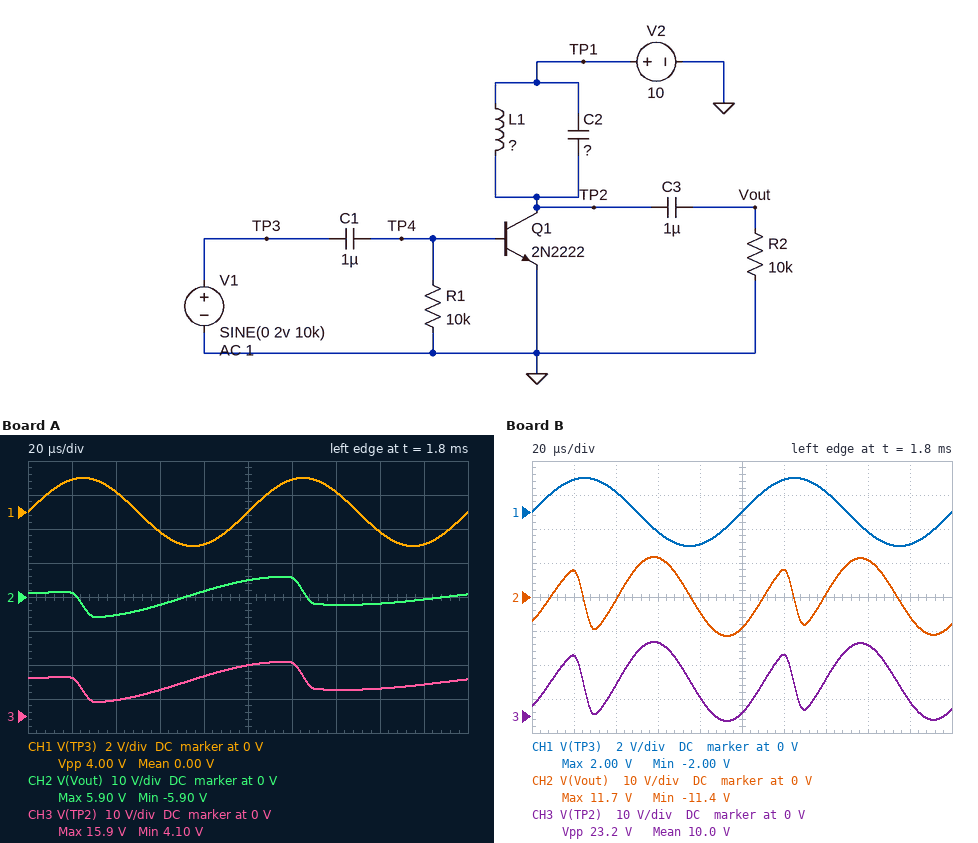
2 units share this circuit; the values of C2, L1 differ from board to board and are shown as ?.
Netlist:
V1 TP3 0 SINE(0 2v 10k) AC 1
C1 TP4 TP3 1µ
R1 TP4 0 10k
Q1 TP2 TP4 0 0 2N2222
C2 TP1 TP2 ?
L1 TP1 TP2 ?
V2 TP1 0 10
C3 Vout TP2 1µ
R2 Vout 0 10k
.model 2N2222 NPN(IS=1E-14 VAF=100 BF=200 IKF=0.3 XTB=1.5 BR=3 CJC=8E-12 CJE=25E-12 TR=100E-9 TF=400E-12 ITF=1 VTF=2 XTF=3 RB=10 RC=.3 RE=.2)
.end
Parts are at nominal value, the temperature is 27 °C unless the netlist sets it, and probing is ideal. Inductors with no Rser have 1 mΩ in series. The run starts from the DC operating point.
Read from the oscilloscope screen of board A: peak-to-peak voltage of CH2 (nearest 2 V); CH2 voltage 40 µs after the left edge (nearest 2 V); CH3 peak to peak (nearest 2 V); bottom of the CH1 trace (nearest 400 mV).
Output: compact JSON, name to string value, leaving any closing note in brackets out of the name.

{"peak-to-peak voltage of CH2": "12 V", "CH2 voltage 40 µs after the left edge": "-6 V", "CH3 peak to peak": "12 V", "bottom of the CH1 trace": "-2.0 V"}
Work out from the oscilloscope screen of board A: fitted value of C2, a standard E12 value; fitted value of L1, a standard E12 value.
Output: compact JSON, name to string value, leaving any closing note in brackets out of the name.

{"fitted value of C2, a standard E12 value": "220 nF", "fitted value of L1, a standard E12 value": "3.9 mH"}
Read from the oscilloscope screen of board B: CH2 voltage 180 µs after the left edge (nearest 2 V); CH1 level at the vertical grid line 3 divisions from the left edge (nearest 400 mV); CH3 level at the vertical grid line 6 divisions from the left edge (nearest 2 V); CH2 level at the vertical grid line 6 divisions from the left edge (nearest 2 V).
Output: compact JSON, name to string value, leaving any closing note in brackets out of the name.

{"CH2 voltage 180 µs after the left edge": "-6 V", "CH1 level at the vertical grid line 3 divisions from the left edge": "-1.2 V", "CH3 level at the vertical grid line 6 divisions from the left edge": "18 V", "CH2 level at the vertical grid line 6 divisions from the left edge": "8 V"}
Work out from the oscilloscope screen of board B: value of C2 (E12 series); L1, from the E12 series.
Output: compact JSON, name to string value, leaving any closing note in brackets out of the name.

{"value of C2": "68 nF", "L1, from the E12 series": "1.8 mH"}
